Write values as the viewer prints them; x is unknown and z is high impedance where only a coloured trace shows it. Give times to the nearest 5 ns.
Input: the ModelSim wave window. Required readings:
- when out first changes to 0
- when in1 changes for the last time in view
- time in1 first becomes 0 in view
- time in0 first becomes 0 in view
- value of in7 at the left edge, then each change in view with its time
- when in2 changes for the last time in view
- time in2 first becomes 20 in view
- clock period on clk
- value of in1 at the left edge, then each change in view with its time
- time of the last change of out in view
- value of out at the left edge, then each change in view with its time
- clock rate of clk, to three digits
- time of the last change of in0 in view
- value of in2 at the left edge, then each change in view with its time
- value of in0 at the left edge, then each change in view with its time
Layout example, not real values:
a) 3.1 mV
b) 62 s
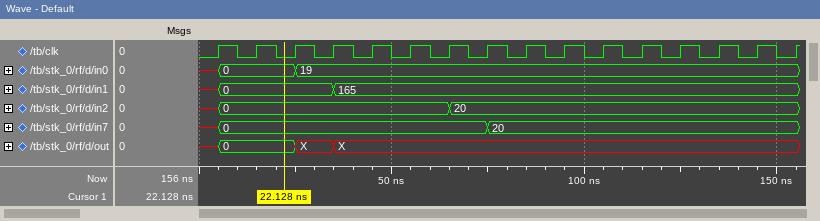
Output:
a) 5 ns
b) 35 ns
c) 5 ns
d) 5 ns
e) x, 0 at 5 ns, 20 at 75 ns
f) 65 ns
g) 65 ns
h) 10 ns
i) x, 0 at 5 ns, 165 at 35 ns
j) 35 ns
k) x, 0 at 5 ns, X at 25 ns, X at 35 ns
l) 100 MHz
m) 25 ns
n) x, 0 at 5 ns, 20 at 65 ns
o) x, 0 at 5 ns, 19 at 25 ns
